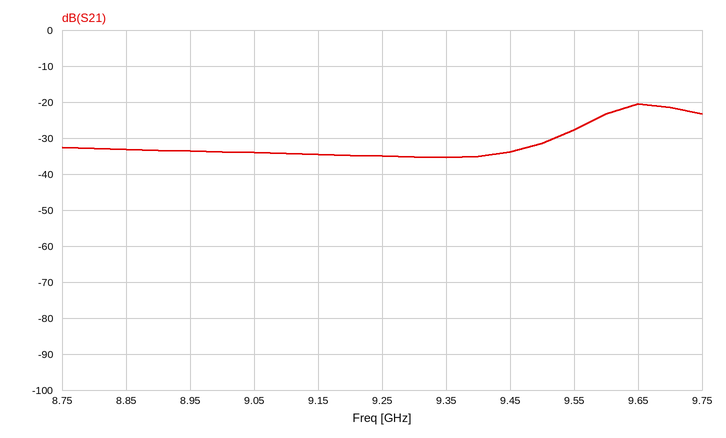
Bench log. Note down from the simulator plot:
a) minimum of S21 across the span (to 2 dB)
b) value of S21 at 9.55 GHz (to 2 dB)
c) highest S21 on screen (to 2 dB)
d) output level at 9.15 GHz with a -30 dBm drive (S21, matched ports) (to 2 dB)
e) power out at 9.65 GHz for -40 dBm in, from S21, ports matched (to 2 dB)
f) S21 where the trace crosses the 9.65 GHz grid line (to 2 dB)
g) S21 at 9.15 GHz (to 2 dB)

-36 dB
-28 dB
-20 dB
-64 dBm
-60 dBm
-20 dB
-34 dB
